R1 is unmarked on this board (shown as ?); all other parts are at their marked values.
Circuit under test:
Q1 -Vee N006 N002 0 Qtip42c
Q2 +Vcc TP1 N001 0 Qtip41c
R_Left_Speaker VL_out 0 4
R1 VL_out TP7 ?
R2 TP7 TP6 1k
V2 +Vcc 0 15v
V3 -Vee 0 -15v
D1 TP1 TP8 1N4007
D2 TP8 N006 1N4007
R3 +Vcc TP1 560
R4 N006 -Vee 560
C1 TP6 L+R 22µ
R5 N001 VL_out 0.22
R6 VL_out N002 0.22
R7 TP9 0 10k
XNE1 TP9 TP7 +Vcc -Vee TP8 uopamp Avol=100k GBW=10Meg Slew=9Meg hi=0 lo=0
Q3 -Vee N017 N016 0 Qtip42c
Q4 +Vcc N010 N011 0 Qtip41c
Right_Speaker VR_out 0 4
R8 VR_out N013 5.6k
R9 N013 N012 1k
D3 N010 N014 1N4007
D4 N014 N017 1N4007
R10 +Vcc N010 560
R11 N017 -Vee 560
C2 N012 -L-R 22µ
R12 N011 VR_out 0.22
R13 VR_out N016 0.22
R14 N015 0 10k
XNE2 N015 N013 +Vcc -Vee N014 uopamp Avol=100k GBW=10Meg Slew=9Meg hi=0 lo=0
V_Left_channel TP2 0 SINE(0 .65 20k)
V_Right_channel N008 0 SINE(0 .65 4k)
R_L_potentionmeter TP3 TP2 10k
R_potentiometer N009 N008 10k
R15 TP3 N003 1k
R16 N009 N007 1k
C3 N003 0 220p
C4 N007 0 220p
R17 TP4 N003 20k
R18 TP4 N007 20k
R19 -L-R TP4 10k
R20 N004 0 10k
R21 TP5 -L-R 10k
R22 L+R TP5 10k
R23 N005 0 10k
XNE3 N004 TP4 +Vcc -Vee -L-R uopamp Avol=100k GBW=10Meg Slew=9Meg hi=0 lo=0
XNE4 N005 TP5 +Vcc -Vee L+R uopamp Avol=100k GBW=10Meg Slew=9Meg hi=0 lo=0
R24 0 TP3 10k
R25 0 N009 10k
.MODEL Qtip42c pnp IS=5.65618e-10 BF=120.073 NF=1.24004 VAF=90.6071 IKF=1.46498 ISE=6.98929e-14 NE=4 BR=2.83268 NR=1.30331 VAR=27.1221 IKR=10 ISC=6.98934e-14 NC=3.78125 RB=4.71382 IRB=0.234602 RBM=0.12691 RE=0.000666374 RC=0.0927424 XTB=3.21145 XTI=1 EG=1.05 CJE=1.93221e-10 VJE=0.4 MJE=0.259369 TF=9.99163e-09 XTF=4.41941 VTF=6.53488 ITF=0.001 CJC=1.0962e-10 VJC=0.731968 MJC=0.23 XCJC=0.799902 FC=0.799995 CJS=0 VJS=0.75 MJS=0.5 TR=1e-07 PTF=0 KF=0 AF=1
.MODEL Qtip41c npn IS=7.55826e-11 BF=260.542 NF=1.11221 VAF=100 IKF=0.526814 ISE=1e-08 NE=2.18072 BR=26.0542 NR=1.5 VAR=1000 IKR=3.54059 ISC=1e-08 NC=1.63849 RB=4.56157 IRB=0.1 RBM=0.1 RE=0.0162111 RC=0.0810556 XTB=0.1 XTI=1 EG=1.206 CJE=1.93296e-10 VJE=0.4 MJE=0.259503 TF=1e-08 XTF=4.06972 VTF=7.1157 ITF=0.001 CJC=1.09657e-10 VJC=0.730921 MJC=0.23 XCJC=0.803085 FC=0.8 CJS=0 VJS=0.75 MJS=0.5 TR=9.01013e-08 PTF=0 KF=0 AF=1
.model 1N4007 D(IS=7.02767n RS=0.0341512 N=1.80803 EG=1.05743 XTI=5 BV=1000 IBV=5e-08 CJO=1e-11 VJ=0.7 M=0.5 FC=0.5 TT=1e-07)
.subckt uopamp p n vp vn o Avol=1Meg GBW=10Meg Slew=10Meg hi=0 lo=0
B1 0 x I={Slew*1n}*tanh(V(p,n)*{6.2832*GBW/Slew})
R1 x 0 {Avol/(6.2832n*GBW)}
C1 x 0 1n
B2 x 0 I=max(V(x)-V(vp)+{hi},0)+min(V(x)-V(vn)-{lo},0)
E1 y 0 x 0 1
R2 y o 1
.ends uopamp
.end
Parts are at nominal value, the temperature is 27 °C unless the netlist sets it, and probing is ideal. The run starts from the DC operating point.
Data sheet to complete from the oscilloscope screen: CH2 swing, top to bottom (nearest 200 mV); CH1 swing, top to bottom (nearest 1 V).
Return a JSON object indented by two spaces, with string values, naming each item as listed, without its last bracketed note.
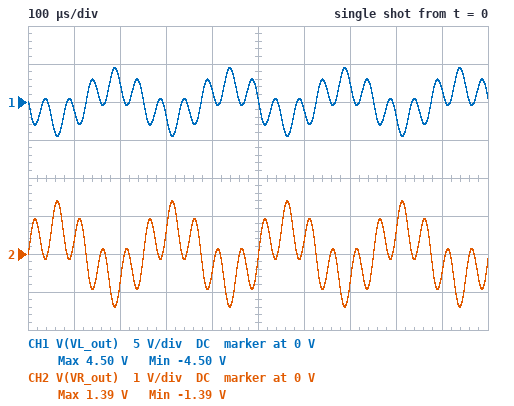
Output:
{
  "CH2 swing, top to bottom": "2.8 V",
  "CH1 swing, top to bottom": "9 V"
}
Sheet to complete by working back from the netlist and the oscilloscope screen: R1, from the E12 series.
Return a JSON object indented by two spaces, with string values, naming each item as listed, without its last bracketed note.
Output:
{
  "R1, from the E12 series": "18 kΩ"
}
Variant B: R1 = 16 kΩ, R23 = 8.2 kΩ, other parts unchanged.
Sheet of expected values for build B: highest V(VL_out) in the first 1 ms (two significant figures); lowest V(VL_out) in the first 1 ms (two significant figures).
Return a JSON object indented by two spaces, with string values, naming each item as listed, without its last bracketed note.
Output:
{
  "highest V(VL_out) in the first 1 ms": "4.0 V",
  "lowest V(VL_out) in the first 1 ms": "-4.0 V"
}
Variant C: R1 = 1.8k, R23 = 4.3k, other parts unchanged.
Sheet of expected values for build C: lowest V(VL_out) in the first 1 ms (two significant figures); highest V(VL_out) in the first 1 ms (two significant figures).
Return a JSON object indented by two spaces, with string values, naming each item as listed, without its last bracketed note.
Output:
{
  "lowest V(VL_out) in the first 1 ms": "-450 mV",
  "highest V(VL_out) in the first 1 ms": "450 mV"
}
